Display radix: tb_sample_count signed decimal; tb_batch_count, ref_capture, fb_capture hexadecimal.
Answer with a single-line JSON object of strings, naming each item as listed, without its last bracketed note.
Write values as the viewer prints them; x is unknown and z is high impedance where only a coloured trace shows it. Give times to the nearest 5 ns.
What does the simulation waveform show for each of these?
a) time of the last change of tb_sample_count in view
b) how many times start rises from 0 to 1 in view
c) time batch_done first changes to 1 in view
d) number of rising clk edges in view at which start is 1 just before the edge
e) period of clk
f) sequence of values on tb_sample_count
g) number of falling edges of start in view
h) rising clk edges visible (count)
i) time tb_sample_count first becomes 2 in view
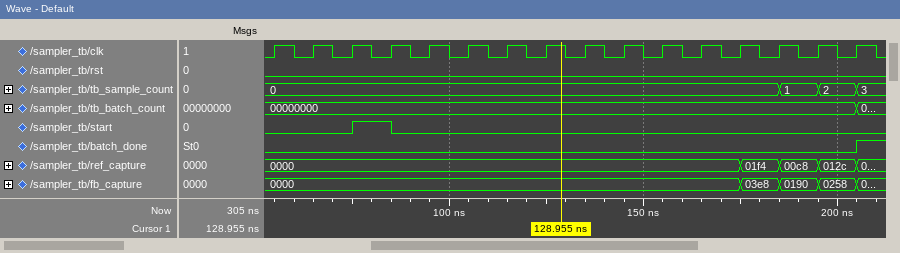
{"time of the last change of tb_sample_count in view": "205 ns", "how many times start rises from 0 to 1 in view": "1", "time batch_done first changes to 1 in view": "205 ns", "number of rising clk edges in view at which start is 1 just before the edge": "1", "period of clk": "10 ns", "sequence of values on tb_sample_count": "0, 1, 2, 3", "number of falling edges of start in view": "1", "rising clk edges visible": "16", "time tb_sample_count first becomes 2 in view": "195 ns"}
